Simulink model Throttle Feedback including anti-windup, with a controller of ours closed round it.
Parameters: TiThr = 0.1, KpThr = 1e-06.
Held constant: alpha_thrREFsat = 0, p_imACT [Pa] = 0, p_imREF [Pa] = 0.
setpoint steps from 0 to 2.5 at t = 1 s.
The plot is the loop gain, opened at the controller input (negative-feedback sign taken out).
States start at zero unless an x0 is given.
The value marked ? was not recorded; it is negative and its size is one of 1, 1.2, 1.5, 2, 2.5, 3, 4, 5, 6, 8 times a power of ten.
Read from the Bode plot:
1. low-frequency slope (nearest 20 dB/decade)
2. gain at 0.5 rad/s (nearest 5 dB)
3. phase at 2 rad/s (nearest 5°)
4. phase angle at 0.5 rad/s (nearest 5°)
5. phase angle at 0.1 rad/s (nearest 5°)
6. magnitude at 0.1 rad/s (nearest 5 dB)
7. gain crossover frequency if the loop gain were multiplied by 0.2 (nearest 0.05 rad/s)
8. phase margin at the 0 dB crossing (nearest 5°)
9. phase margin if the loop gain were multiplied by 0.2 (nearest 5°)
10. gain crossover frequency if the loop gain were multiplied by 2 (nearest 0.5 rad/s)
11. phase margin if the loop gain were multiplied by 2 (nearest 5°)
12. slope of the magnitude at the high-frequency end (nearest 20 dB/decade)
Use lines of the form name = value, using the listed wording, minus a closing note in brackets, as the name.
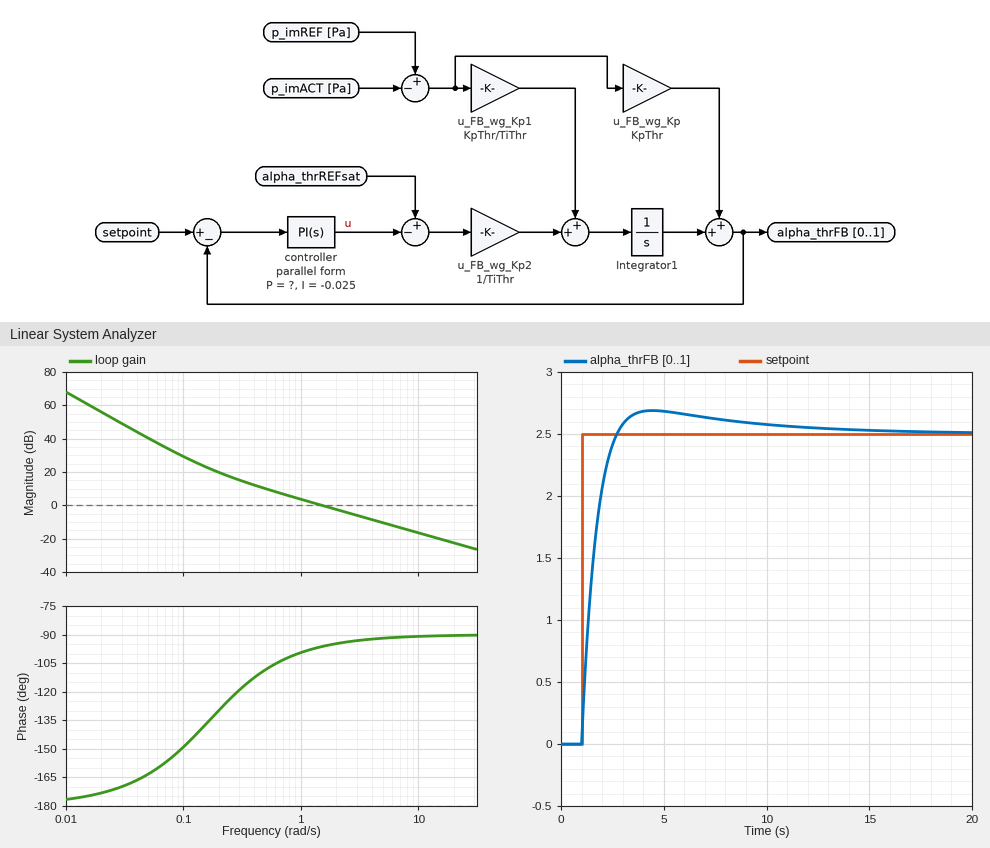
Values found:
low-frequency slope = -40 dB/decade
gain at 0.5 rad/s = 10 dB
phase at 2 rad/s = -95°
phase angle at 0.5 rad/s = -110°
phase angle at 0.1 rad/s = -150°
magnitude at 0.1 rad/s = 30 dB
gain crossover frequency if the loop gain were multiplied by 0.2 = 0.35 rad/s
phase margin at the 0 dB crossing = 85°
phase margin if the loop gain were multiplied by 0.2 = 65°
gain crossover frequency if the loop gain were multiplied by 2 = 3.0 rad/s
phase margin if the loop gain were multiplied by 2 = 85°
slope of the magnitude at the high-frequency end = -20 dB/decade
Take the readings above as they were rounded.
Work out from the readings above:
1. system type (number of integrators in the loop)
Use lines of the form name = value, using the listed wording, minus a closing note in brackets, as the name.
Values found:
system type = 2
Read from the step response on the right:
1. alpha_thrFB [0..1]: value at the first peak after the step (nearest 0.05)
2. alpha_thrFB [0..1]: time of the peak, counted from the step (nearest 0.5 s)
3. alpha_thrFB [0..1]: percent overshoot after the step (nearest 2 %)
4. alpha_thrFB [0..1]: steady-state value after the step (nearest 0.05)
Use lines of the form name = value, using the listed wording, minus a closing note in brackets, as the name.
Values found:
alpha_thrFB [0..1]: value at the first peak after the step = 2.70
alpha_thrFB [0..1]: time of the peak, counted from the step = 3.5 s
alpha_thrFB [0..1]: percent overshoot after the step = 8 %
alpha_thrFB [0..1]: steady-state value after the step = 2.50
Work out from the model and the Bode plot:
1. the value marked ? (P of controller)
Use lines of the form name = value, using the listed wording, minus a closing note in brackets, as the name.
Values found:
the value marked ? = -0.15
